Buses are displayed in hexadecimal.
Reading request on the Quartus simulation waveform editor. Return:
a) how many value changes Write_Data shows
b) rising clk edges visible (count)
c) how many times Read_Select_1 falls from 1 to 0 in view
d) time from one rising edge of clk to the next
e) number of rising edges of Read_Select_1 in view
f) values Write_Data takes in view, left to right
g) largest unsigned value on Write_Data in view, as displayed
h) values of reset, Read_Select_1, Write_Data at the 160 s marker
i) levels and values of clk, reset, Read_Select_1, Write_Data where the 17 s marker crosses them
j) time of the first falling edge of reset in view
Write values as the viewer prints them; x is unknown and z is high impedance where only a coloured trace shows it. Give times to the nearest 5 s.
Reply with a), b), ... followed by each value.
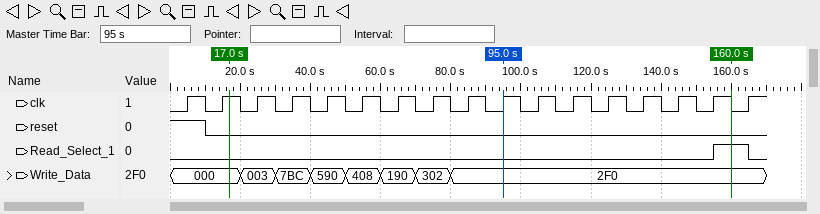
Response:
a) 7
b) 17
c) 1
d) 10 s
e) 1
f) 000, 003, 7BC, 590, 408, 190, 302, 2F0
g) 7BC
h) reset=0, Read_Select_1=1, Write_Data=2F0
i) clk=1, reset=0, Read_Select_1=0, Write_Data=000
j) 10 s
